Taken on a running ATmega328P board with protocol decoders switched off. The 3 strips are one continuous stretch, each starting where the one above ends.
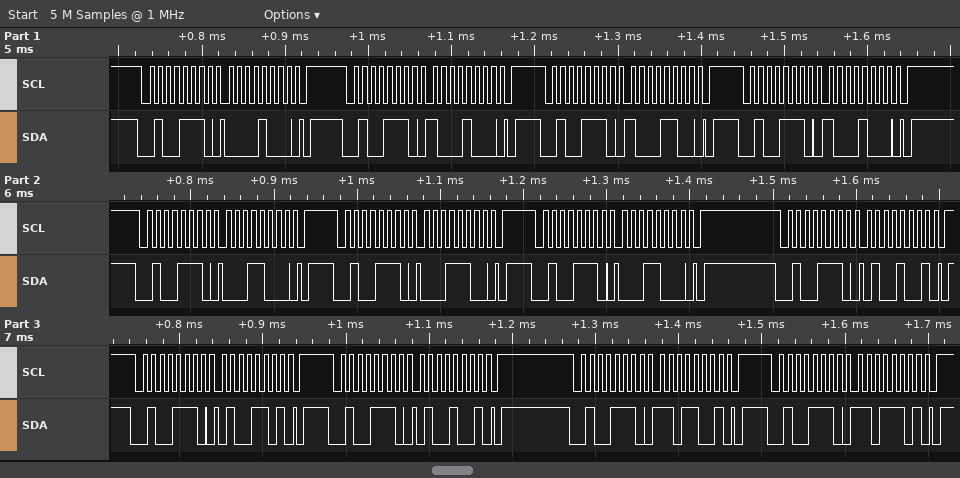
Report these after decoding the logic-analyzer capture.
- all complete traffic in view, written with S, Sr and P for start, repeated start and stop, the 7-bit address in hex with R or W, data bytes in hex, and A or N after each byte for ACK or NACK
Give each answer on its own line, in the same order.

S 27W A 08 A P S 27W A 88 A P S 27W A 8C A P S 27W A 88 A P S 27W A 18 A P S 27W A 1C A P S 27W A 18 A P S 27W A 49 A P S 27W A 4D A P S 27W A 49 A P S 27W A D9 A P S 27W A DD A P
